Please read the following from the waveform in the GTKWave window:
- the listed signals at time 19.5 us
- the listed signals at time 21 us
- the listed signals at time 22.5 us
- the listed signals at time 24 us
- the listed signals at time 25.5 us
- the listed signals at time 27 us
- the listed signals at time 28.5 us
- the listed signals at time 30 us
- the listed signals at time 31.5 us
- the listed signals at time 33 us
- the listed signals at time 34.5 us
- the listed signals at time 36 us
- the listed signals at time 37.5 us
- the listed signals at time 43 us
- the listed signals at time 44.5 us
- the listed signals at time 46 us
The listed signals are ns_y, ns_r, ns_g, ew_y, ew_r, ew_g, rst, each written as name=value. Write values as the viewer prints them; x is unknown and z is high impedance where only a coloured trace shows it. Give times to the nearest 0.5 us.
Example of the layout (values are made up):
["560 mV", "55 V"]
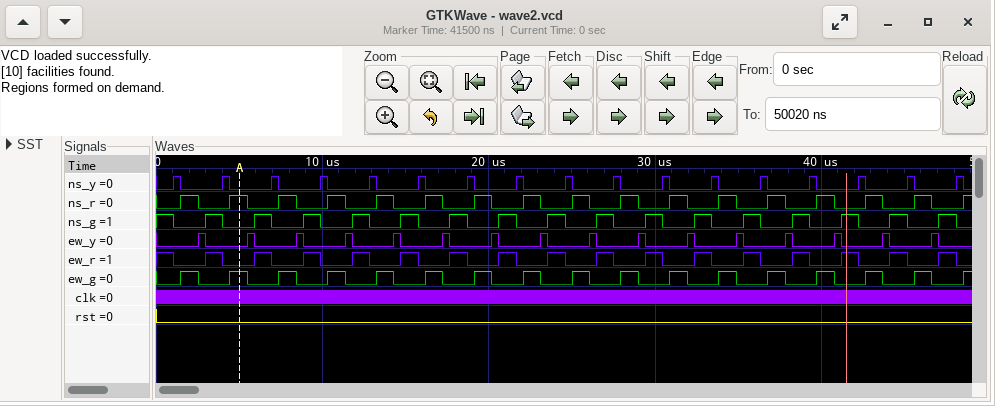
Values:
["ns_y=0, ns_r=1, ns_g=0, ew_y=0, ew_r=0, ew_g=1, rst=0", "ns_y=0, ns_r=0, ns_g=1, ew_y=0, ew_r=1, ew_g=0, rst=0", "ns_y=0, ns_r=1, ns_g=0, ew_y=0, ew_r=0, ew_g=1, rst=0", "ns_y=0, ns_r=0, ns_g=1, ew_y=0, ew_r=1, ew_g=0, rst=0", "ns_y=0, ns_r=1, ns_g=0, ew_y=0, ew_r=0, ew_g=1, rst=0", "ns_y=0, ns_r=0, ns_g=1, ew_y=0, ew_r=1, ew_g=0, rst=0", "ns_y=0, ns_r=1, ns_g=0, ew_y=0, ew_r=0, ew_g=1, rst=0", "ns_y=0, ns_r=0, ns_g=1, ew_y=0, ew_r=1, ew_g=0, rst=0", "ns_y=0, ns_r=1, ns_g=0, ew_y=0, ew_r=0, ew_g=1, rst=0", "ns_y=0, ns_r=0, ns_g=1, ew_y=0, ew_r=1, ew_g=0, rst=0", "ns_y=0, ns_r=1, ns_g=0, ew_y=0, ew_r=0, ew_g=1, rst=0", "ns_y=0, ns_r=0, ns_g=1, ew_y=0, ew_r=1, ew_g=0, rst=0", "ns_y=0, ns_r=1, ns_g=0, ew_y=0, ew_r=0, ew_g=1, rst=0", "ns_y=0, ns_r=1, ns_g=0, ew_y=0, ew_r=0, ew_g=1, rst=0", "ns_y=0, ns_r=0, ns_g=1, ew_y=0, ew_r=1, ew_g=0, rst=0", "ns_y=0, ns_r=1, ns_g=0, ew_y=0, ew_r=0, ew_g=1, rst=0"]
